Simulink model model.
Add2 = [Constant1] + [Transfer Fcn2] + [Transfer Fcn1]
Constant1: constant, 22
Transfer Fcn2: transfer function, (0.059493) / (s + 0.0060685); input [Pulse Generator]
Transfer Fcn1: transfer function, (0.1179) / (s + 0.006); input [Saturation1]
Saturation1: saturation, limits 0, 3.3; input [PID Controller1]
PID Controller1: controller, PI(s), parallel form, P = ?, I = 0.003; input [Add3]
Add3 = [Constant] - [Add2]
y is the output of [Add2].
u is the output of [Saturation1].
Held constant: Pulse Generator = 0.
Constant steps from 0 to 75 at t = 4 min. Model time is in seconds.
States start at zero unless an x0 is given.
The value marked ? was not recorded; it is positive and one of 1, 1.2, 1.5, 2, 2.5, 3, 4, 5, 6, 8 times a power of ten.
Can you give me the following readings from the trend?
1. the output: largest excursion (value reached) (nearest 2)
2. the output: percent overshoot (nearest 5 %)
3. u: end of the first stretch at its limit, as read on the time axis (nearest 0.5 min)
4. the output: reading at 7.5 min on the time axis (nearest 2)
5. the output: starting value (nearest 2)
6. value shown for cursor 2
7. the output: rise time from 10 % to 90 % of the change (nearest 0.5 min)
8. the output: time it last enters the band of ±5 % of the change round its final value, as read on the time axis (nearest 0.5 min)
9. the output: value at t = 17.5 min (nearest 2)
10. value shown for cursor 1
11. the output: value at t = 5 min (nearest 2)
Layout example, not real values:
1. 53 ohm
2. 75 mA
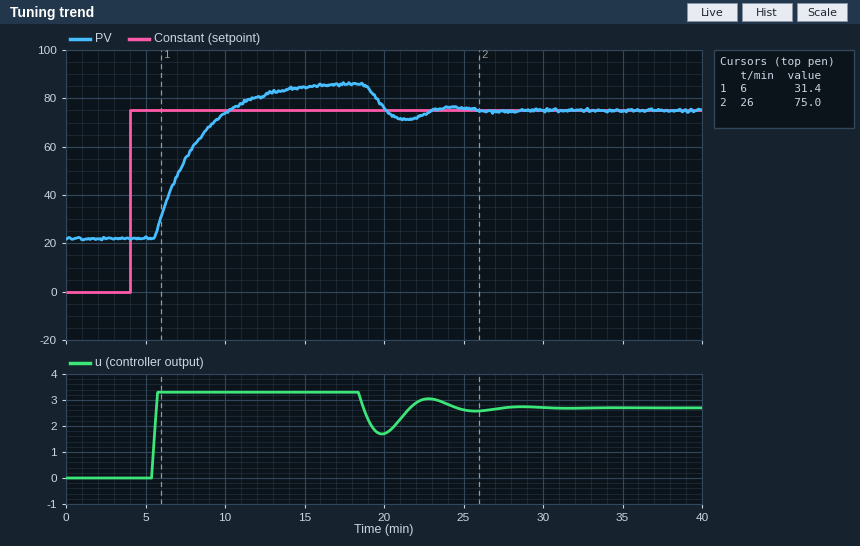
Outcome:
1. 86
2. 20 %
3. 5.5 min
4. 54
5. 22
6. 75.0
7. 3.5 min
8. 22.0 min
9. 86
10. 31.4
11. 22
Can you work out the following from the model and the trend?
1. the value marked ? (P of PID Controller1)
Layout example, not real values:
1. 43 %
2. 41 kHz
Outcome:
1. 0.05
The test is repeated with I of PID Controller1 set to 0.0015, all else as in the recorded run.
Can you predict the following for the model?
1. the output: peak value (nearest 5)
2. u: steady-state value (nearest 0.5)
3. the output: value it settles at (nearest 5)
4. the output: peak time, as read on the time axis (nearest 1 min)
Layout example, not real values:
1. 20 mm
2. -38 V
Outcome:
1. 85
2. 2.5
3. 75
4. 16 min
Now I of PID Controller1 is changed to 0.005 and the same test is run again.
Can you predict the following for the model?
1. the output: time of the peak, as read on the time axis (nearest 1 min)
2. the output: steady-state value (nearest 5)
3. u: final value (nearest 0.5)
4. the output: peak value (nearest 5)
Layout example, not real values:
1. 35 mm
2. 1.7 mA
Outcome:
1. 19 min
2. 75
3. 2.5
4. 85
